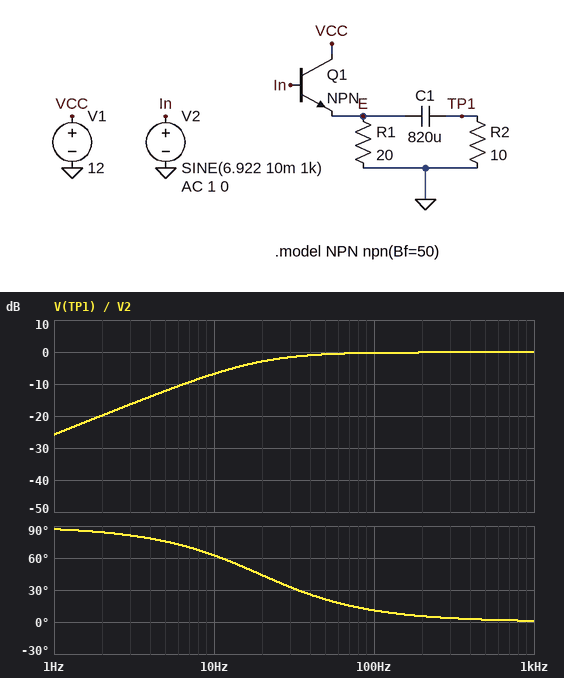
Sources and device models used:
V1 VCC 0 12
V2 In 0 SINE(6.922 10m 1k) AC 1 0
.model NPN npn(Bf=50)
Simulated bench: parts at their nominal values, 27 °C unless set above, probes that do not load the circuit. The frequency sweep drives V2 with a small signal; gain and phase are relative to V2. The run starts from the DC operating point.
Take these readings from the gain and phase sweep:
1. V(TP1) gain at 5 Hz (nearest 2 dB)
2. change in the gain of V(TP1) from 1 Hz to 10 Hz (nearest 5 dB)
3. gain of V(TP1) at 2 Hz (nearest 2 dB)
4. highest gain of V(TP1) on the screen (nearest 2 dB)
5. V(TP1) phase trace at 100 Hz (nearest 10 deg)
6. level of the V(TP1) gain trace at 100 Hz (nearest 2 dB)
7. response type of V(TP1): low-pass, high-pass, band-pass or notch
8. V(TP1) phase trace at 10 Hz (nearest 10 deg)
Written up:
-12 dB
20 dB
-20 dB
0 dB
10 deg
0 dB
high-pass
60 deg
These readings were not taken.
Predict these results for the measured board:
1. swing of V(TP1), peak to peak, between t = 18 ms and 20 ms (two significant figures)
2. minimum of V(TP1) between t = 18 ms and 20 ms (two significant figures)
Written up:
20 mV
-9.9 mV
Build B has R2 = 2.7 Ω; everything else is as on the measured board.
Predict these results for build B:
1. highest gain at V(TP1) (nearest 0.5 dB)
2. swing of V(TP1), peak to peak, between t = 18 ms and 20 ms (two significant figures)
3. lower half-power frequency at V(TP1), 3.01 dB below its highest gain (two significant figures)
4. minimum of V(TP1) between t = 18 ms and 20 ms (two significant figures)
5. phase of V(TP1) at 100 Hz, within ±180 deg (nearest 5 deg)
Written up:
-0.5 dB
19 mV
70 Hz
-9.6 mV
35 deg
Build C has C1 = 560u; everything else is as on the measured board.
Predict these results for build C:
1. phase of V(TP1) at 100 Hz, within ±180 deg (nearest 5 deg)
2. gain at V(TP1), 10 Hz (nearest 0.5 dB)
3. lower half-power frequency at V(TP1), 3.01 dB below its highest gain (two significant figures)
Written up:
15 deg
-9.5 dB
28 Hz
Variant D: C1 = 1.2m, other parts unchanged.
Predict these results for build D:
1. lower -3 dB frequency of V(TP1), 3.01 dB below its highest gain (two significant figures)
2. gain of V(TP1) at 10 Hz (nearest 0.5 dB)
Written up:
13 Hz
-4.5 dB
